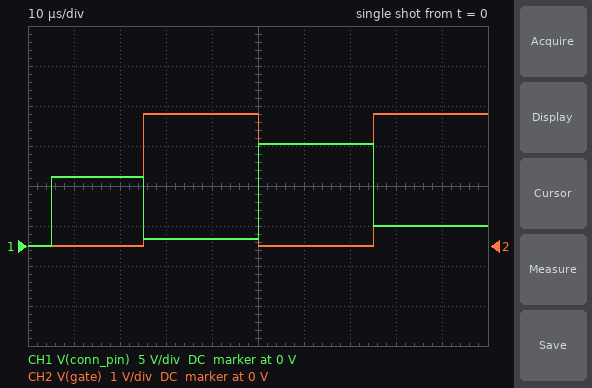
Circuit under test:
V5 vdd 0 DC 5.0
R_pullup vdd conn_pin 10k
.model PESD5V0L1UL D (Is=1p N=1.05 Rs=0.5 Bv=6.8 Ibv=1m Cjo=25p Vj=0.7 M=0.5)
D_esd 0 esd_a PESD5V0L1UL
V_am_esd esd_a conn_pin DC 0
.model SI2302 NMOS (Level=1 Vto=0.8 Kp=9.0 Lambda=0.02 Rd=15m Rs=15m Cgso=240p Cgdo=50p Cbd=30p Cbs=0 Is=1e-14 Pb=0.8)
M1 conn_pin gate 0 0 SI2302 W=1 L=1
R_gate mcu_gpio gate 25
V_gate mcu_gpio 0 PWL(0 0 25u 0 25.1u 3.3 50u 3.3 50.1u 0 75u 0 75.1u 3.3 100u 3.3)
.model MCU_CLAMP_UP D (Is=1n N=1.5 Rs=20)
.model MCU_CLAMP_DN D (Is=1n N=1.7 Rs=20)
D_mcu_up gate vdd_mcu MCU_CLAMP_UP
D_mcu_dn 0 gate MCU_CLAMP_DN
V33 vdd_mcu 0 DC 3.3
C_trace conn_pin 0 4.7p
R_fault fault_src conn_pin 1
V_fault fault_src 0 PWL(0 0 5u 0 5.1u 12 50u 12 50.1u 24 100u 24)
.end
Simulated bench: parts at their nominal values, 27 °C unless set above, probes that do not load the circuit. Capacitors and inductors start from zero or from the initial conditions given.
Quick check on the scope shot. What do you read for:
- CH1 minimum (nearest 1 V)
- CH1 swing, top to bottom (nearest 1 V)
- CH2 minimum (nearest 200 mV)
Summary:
0 V
13 V
0 V
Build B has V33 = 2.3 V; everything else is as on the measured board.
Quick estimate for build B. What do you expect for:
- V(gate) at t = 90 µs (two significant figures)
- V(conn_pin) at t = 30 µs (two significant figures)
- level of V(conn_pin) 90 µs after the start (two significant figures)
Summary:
3.1 V
1.0 V
4.6 V
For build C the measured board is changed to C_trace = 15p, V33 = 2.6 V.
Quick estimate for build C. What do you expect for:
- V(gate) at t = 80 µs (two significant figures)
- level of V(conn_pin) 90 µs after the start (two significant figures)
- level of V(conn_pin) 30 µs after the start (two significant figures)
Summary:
3.2 V
2.9 V
950 mV
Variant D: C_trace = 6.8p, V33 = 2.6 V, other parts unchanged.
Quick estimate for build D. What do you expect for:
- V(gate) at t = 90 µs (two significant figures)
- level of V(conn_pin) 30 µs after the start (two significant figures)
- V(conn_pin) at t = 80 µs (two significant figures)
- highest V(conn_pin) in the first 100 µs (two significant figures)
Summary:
3.2 V
950 mV
2.9 V
13 V
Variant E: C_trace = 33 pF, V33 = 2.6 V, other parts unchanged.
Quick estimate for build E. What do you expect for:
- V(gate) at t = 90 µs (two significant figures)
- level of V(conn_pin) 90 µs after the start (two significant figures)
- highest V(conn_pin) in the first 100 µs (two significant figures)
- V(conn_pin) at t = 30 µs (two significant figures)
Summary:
3.2 V
2.9 V
13 V
950 mV
